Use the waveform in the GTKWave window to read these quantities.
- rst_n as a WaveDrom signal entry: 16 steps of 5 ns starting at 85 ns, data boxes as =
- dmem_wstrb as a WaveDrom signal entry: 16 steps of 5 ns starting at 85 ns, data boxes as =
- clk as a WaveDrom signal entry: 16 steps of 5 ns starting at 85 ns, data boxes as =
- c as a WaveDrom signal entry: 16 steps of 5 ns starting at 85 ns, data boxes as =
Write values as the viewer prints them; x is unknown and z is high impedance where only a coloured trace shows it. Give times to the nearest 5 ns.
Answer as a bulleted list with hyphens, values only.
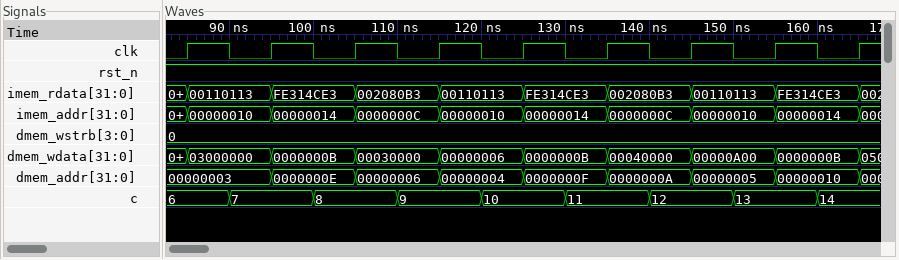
- {name: 'rst_n', wave: '1...............'}
- {name: 'dmem_wstrb', wave: '=...............', data: '0'}
- {name: 'clk', wave: '1010101010101010'}
- {name: 'c', wave: '==.=.=.=.=.=.=.=', data: '6 7 8 9 10 11 12 13 14'}
